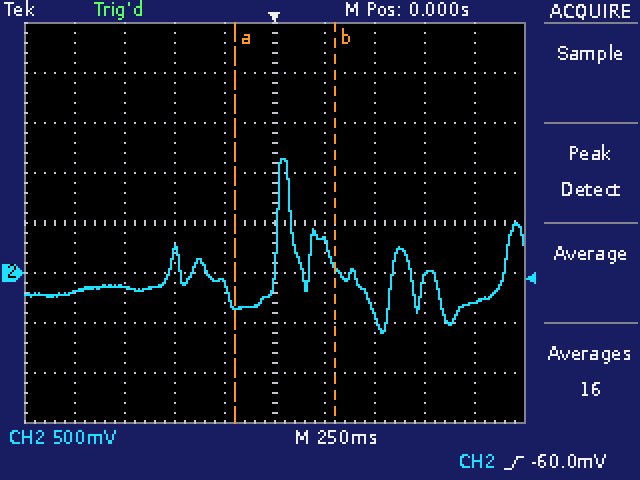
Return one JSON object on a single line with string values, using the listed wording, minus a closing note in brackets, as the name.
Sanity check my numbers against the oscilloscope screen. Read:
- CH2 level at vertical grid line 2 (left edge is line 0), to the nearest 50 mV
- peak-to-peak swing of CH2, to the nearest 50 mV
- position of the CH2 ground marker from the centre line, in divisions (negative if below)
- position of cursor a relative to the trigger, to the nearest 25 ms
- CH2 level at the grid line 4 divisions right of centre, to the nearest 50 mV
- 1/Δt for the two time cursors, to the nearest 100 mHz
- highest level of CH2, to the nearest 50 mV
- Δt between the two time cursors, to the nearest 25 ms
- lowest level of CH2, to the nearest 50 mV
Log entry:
{"CH2 level at vertical grid line 2 (left edge is line 0), to the nearest 50 mV": "-150 mV", "peak-to-peak swing of CH2, to the nearest 50 mV": "1.75 V", "position of the CH2 ground marker from the centre line, in divisions": "-1.0 div", "position of cursor a relative to the trigger, to the nearest 25 ms": "-200 ms", "CH2 level at the grid line 4 divisions right of centre, to the nearest 50 mV": "-300 mV", "1/Δt for the two time cursors, to the nearest 100 mHz": "2.0 Hz", "highest level of CH2, to the nearest 50 mV": "1.15 V", "Δt between the two time cursors, to the nearest 25 ms": "500 ms", "lowest level of CH2, to the nearest 50 mV": "-600 mV"}
